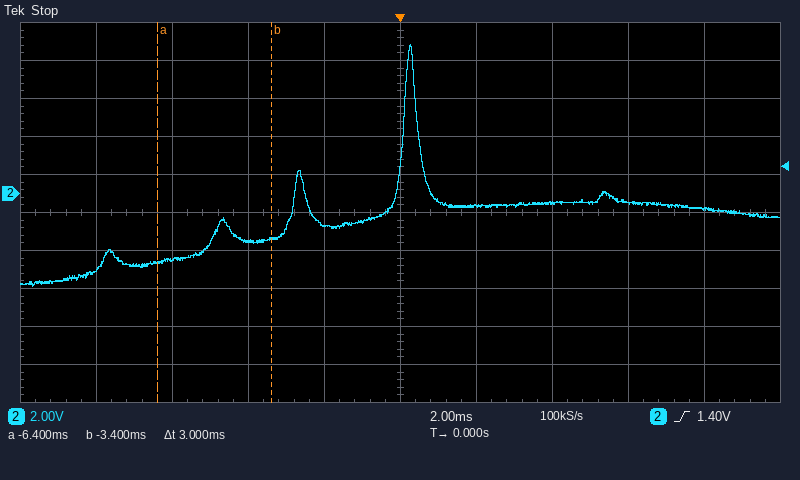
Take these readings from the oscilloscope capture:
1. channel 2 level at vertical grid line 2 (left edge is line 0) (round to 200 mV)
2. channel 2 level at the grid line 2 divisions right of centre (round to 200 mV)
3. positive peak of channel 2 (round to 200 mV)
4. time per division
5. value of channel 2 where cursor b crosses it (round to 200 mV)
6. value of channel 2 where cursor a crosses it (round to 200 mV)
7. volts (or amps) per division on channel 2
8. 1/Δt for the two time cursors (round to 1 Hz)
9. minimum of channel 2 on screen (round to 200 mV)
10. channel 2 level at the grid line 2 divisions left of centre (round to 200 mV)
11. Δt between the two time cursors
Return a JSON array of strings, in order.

["-3.4 V", "-400 mV", "7.8 V", "2 ms", "-2.4 V", "-3.6 V", "2 V", "333 Hz", "-4.8 V", "-2.4 V", "3 ms"]
